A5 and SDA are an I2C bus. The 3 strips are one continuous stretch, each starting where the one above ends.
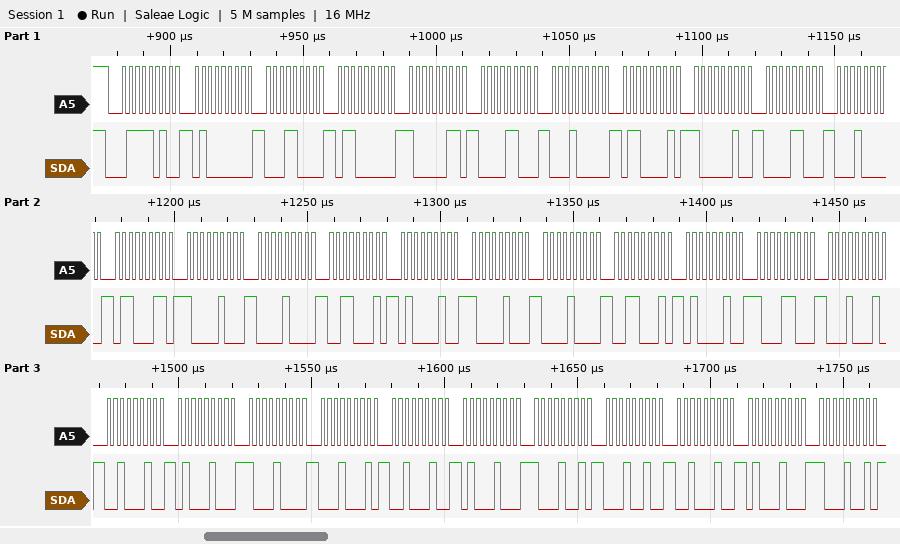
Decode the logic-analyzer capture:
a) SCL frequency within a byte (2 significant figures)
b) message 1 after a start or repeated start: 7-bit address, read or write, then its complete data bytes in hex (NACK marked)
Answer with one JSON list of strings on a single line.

["400 kHz", "0x3D write: 40 18 60 83 0C 10 61 82 0C 10 63 84 08 31 42 84 08 31 42 8C 11 22 44 88 11 22 44 89 12 22 44 89"]
